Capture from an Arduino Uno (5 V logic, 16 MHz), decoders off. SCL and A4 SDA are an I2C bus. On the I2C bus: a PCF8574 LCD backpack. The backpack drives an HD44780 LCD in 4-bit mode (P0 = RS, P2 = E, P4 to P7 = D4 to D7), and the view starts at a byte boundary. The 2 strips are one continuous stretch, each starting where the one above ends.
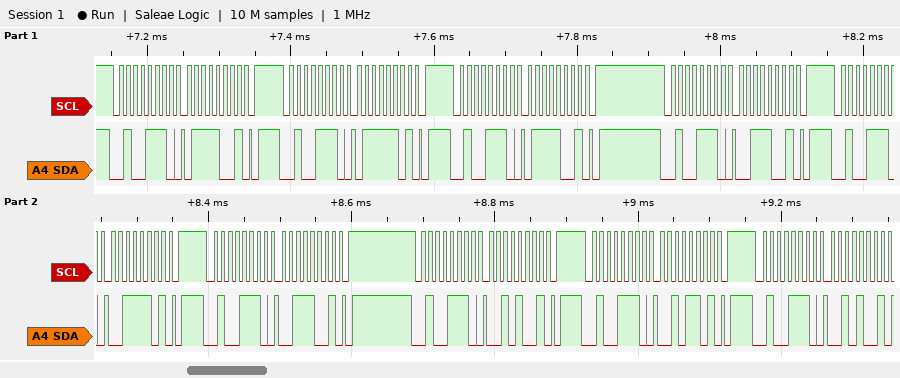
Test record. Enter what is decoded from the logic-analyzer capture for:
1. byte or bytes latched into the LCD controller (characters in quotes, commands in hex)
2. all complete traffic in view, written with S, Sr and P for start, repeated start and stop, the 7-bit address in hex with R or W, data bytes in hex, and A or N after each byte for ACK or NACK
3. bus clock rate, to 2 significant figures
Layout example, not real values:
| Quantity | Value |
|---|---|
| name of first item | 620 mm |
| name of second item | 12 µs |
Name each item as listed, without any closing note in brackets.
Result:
| Quantity | Value |
|---|---|
| byte or bytes latched into the LCD controller | 's' |
| all complete traffic in view, written with S, Sr and P for start, repeated start and stop, the 7-bit address in hex with R or W, data bytes in hex, and A or N after each byte for ACK or NACK | S 27W A 79 A P S 27W A 7D A P S 27W A 79 A P S 27W A 39 A P S 27W A 3D A P S 27W A 39 A P S 27W A 29 A P S 27W A 2D A P S 27W A 29 A |
| bus clock rate, to 2 significant figures | 100 kHz |
